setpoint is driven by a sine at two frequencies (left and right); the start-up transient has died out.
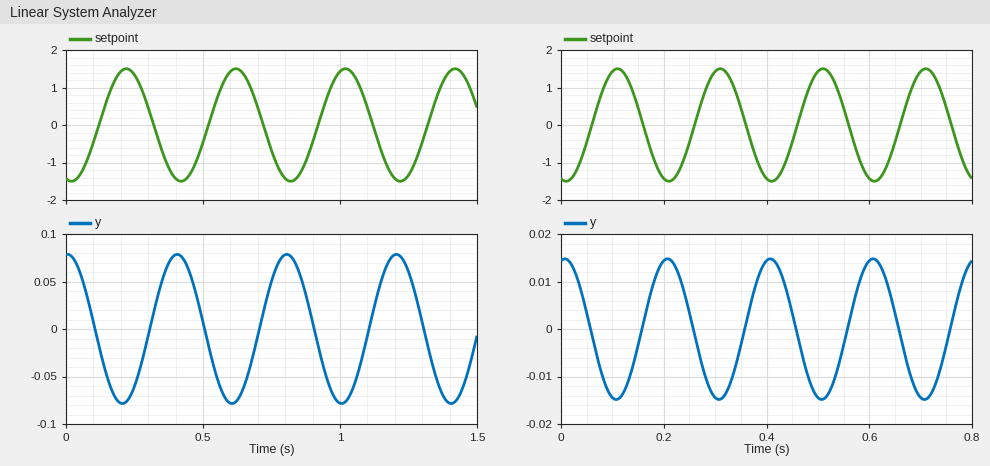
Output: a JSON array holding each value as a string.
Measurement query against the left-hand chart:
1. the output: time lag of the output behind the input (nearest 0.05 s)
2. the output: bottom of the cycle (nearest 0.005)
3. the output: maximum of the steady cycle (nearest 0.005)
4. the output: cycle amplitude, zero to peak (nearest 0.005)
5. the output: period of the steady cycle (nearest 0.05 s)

["0.20 s", "-0.080", "0.080", "0.080", "0.40 s"]
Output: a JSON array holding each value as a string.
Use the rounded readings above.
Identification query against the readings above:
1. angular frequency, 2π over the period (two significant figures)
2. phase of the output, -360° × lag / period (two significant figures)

["16 rad/s", "-180°"]
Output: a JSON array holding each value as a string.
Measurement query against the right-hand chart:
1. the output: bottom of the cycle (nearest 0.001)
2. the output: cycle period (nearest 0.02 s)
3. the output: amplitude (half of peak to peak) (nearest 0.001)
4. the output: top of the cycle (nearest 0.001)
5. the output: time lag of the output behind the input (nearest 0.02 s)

["-0.015", "0.20 s", "0.015", "0.015", "0.10 s"]
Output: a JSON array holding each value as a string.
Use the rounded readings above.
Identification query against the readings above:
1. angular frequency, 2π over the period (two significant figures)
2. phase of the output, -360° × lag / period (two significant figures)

["31 rad/s", "-180°"]
